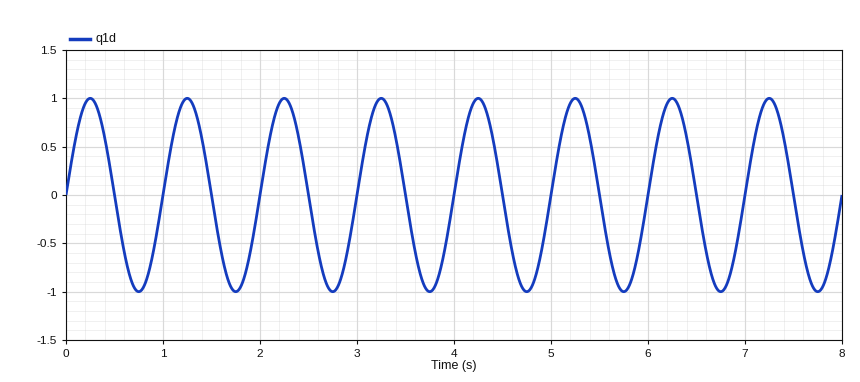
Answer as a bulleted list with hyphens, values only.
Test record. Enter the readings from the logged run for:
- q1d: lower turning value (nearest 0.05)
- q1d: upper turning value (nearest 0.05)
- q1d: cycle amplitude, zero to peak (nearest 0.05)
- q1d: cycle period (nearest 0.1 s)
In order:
- -1.00
- 1.00
- 1.00
- 1.0 s
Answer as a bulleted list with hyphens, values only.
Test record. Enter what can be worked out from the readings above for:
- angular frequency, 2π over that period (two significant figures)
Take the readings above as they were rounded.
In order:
- 6.3 rad/s
